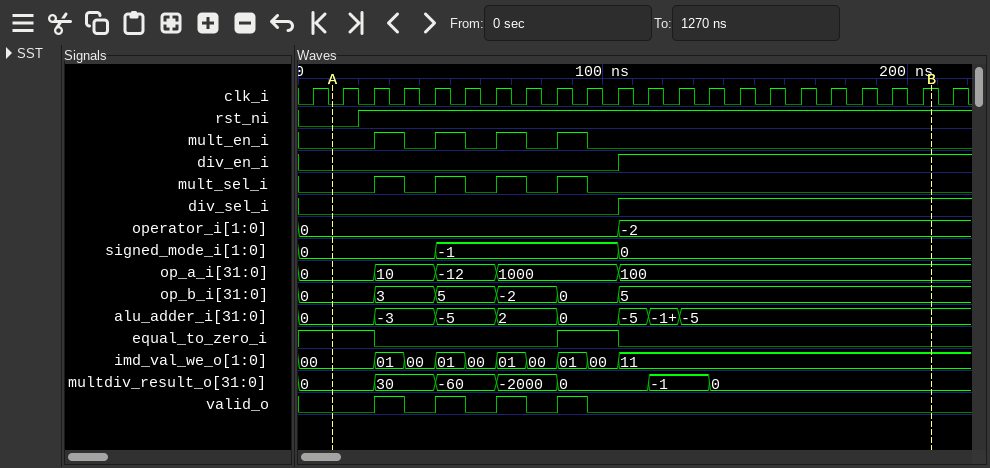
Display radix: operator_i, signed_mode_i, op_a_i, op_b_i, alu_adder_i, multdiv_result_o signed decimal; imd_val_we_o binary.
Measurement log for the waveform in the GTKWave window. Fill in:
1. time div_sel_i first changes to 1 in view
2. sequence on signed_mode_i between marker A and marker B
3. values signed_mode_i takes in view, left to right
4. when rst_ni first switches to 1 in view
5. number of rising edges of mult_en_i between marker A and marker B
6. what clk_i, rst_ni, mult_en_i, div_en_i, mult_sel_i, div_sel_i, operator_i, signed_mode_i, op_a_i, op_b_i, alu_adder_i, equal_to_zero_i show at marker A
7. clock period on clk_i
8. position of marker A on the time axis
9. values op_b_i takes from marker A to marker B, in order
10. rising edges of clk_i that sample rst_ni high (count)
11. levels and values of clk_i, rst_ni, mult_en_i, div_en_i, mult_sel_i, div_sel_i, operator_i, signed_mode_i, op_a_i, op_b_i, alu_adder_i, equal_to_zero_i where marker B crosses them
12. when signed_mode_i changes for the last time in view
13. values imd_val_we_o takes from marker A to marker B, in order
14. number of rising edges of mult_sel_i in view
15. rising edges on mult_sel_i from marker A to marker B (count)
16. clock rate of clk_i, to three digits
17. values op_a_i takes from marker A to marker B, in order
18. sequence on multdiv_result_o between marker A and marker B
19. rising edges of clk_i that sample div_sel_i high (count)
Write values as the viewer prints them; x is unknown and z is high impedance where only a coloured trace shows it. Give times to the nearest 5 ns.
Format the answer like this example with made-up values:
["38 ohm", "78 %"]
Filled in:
["105 ns", "0, -1, 0", "0, -1, 0", "20 ns", "4", "clk_i=0, rst_ni=0, mult_en_i=0, div_en_i=0, mult_sel_i=0, div_sel_i=0, operator_i=0, signed_mode_i=0, op_a_i=0, op_b_i=0, alu_adder_i=0, equal_to_zero_i=1", "10 ns", "10 ns", "0, 3, 5, -2, 0, 5", "20", "clk_i=1, rst_ni=1, mult_en_i=0, div_en_i=1, mult_sel_i=0, div_sel_i=1, operator_i=-2, signed_mode_i=0, op_a_i=100, op_b_i=5, alu_adder_i=-5, equal_to_zero_i=0", "105 ns", "00, 01, 00, 01, 00, 01, 00, 01, 00, 11", "4", "4", "100 MHz", "0, 10, -12, 1000, 100", "0, 30, -60, -2000, 0, -1, 0", "11"]
